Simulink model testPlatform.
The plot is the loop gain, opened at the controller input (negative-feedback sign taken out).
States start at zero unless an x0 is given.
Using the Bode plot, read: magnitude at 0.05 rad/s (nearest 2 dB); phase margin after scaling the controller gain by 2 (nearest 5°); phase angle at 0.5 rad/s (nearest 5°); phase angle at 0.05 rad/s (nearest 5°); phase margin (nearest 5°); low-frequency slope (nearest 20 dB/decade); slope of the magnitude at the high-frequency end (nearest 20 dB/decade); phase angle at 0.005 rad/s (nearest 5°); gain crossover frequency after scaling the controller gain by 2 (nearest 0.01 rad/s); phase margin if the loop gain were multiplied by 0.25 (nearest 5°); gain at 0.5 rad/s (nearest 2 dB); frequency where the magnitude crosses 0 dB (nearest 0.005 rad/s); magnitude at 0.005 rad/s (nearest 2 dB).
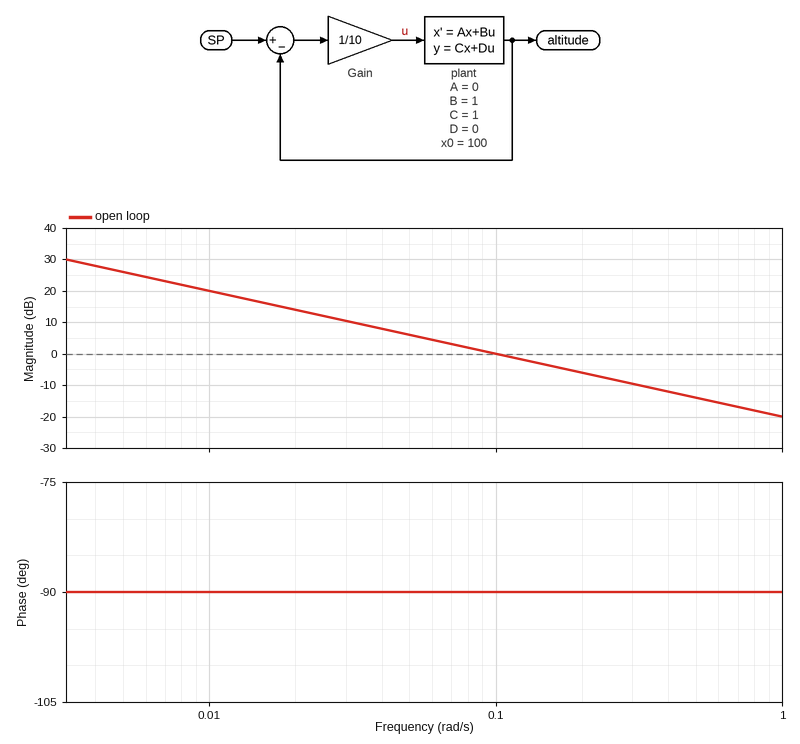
6 dB
90°
-90°
-90°
90°
-20 dB/decade
-20 dB/decade
-90°
0.20 rad/s
90°
-14 dB
0.100 rad/s
26 dB
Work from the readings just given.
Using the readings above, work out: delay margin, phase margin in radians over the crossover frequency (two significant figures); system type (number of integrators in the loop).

16 s
1
